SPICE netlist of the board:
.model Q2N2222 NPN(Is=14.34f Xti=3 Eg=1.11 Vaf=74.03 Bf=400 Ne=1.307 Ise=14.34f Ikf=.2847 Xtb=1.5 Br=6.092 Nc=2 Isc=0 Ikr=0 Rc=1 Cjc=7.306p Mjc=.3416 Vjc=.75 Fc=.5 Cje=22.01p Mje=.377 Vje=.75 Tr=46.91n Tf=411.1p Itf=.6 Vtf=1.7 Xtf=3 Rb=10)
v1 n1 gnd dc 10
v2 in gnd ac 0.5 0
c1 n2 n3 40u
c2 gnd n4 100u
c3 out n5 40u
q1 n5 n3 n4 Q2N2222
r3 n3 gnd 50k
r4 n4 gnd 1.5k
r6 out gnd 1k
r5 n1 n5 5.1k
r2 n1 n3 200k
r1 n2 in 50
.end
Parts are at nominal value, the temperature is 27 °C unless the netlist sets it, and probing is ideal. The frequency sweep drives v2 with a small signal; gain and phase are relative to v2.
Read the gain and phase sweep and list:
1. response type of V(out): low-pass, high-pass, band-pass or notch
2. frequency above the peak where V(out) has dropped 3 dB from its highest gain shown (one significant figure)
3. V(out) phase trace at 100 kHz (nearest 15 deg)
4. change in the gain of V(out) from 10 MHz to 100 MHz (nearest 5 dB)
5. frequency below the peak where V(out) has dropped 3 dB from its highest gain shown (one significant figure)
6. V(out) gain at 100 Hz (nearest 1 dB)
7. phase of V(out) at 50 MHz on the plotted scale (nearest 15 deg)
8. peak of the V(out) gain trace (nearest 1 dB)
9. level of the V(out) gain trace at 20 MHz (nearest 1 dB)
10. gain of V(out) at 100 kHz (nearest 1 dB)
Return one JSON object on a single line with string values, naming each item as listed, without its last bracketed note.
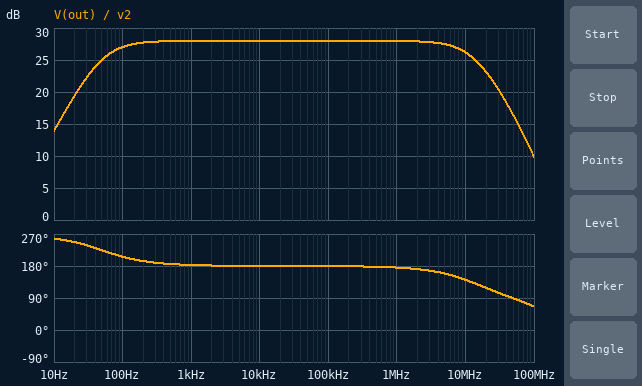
{"response type of V(out): low-pass, high-pass, band-pass or notch": "band-pass", "frequency above the peak where V(out) has dropped 3 dB from its highest gain shown": "10 MHz", "V(out) phase trace at 100 kHz": "180 deg", "change in the gain of V(out) from 10 MHz to 100 MHz": "-15 dB", "frequency below the peak where V(out) has dropped 3 dB from its highest gain shown": "50 Hz", "V(out) gain at 100 Hz": "27 dB", "phase of V(out) at 50 MHz on the plotted scale": "90 deg", "peak of the V(out) gain trace": "28 dB", "level of the V(out) gain trace at 20 MHz": "23 dB", "gain of V(out) at 100 kHz": "28 dB"}
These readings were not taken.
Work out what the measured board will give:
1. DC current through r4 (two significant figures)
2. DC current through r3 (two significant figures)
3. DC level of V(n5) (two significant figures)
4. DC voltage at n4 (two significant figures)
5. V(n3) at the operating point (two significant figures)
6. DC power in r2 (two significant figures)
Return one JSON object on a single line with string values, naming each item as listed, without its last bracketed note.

{"DC current through r4": "800 µA", "DC current through r3": "37 µA", "DC level of V(n5)": "6.0 V", "DC voltage at n4": "1.2 V", "V(n3) at the operating point": "1.8 V", "DC power in r2": "330 µW"}
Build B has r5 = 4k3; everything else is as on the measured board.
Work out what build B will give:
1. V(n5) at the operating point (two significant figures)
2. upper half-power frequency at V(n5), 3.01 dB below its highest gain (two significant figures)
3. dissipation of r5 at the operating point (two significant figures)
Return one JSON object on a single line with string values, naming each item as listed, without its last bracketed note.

{"V(n5) at the operating point": "6.6 V", "upper half-power frequency at V(n5), 3.01 dB below its highest gain": "15 MHz", "dissipation of r5 at the operating point": "2.7 mW"}
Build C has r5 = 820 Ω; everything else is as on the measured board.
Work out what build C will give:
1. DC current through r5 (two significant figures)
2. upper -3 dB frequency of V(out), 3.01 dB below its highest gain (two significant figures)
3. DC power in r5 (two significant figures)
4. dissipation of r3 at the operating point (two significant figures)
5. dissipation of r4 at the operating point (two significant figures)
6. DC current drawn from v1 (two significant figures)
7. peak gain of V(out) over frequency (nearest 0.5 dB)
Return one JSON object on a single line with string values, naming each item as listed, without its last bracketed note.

{"DC current through r5": "800 µA", "upper -3 dB frequency of V(out), 3.01 dB below its highest gain": "24 MHz", "DC power in r5": "520 µW", "dissipation of r3 at the operating point": "68 µW", "dissipation of r4 at the operating point": "960 µW", "DC current drawn from v1": "840 µA", "peak gain of V(out) over frequency": "22.5 dB"}
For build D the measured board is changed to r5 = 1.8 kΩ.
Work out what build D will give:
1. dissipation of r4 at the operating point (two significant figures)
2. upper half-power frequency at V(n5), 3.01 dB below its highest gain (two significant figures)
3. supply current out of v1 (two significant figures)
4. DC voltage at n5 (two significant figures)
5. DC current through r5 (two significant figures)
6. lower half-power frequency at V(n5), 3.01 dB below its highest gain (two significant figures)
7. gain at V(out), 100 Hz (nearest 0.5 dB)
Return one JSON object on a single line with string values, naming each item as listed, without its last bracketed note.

{"dissipation of r4 at the operating point": "960 µW", "upper half-power frequency at V(n5), 3.01 dB below its highest gain": "19 MHz", "supply current out of v1": "840 µA", "DC voltage at n5": "8.6 V", "DC current through r5": "800 µA", "lower half-power frequency at V(n5), 3.01 dB below its highest gain": "50 Hz", "gain at V(out), 100 Hz": "25.0 dB"}
